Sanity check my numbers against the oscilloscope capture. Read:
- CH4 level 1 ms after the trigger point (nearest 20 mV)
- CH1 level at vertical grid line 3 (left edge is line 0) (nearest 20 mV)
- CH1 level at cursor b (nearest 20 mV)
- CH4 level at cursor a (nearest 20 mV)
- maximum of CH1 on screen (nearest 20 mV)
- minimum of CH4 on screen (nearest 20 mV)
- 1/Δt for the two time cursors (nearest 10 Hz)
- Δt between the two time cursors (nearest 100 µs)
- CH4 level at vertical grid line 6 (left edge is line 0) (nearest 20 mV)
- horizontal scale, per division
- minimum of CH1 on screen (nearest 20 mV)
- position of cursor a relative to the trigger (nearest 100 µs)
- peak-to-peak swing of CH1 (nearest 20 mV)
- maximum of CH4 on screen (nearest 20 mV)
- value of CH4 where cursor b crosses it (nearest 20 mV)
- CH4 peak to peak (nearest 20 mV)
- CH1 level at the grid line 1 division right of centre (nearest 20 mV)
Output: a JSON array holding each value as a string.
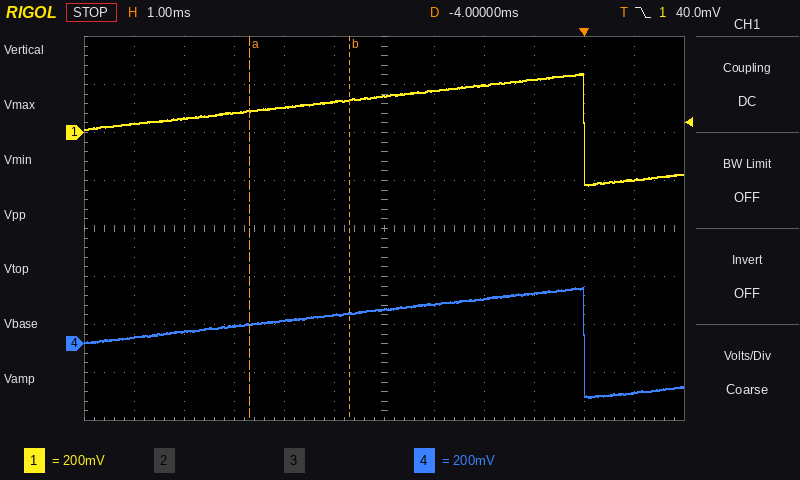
["-200 mV", "80 mV", "140 mV", "80 mV", "240 mV", "-220 mV", "500 Hz", "2.0 ms", "140 mV", "1 ms", "-220 mV", "-6.7 ms", "460 mV", "240 mV", "120 mV", "460 mV", "180 mV"]
